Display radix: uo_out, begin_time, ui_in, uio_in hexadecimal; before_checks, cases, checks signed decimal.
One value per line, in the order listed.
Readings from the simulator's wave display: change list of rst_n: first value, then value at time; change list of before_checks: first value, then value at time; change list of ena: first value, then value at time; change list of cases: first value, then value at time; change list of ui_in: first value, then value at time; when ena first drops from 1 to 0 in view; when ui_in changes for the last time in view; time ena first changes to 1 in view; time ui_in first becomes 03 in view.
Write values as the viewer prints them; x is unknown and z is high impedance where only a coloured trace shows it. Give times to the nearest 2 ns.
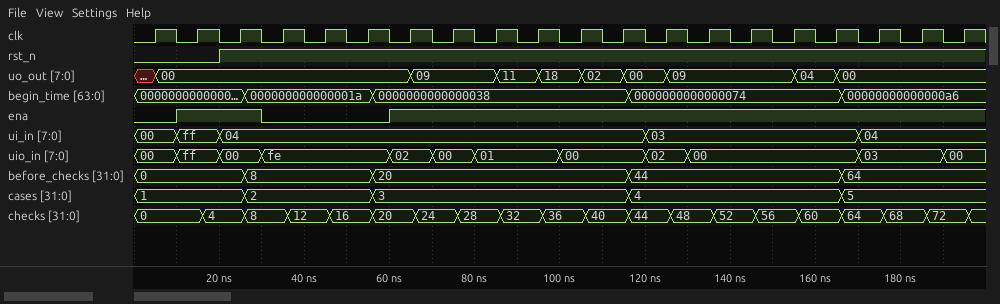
0, 1 at 20 ns
0, 8 at 26 ns, 20 at 56 ns, 44 at 116 ns, 64 at 166 ns
0, 1 at 10 ns, 0 at 30 ns, 1 at 60 ns
1, 2 at 26 ns, 3 at 56 ns, 4 at 116 ns, 5 at 166 ns
00, ff at 10 ns, 04 at 20 ns, 03 at 120 ns, 04 at 170 ns
30 ns
170 ns
10 ns
120 ns
